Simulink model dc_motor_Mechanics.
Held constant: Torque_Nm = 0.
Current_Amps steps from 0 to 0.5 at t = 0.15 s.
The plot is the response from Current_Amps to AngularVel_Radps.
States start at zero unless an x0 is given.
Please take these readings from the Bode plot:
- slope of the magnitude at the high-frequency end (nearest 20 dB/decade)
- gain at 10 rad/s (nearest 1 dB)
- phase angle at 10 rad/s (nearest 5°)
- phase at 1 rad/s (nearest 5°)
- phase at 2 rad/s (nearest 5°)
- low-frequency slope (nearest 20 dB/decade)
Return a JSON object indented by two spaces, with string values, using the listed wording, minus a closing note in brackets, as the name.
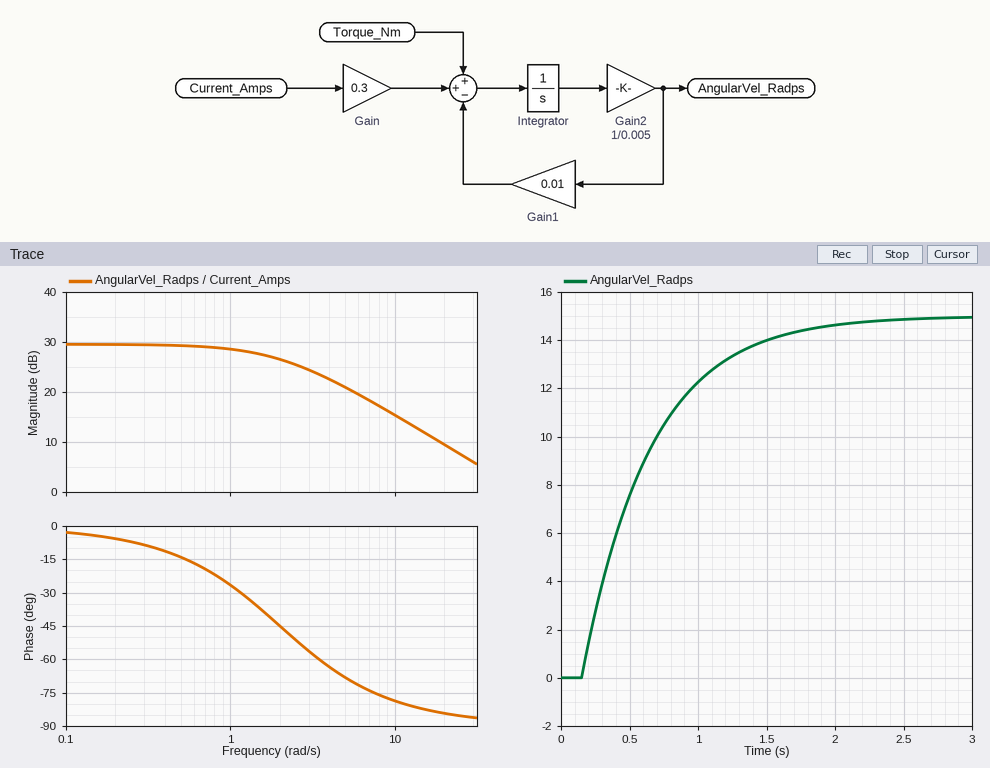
{
  "slope of the magnitude at the high-frequency end": "-20 dB/decade",
  "gain at 10 rad/s": "15 dB",
  "phase angle at 10 rad/s": "-80°",
  "phase at 1 rad/s": "-25°",
  "phase at 2 rad/s": "-45°",
  "low-frequency slope": "0 dB/decade"
}
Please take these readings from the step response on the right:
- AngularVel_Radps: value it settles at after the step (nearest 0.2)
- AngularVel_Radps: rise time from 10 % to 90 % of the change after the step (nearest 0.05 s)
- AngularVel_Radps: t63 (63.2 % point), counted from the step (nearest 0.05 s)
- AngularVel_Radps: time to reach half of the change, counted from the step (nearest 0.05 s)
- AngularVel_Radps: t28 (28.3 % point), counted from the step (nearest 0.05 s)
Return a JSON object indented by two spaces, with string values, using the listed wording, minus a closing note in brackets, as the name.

{
  "AngularVel_Radps: value it settles at after the step": "15.0",
  "AngularVel_Radps: rise time from 10 % to 90 % of the change after the step": "1.10 s",
  "AngularVel_Radps: t63 (63.2 % point), counted from the step": "0.50 s",
  "AngularVel_Radps: time to reach half of the change, counted from the step": "0.35 s",
  "AngularVel_Radps: t28 (28.3 % point), counted from the step": "0.15 s"
}
